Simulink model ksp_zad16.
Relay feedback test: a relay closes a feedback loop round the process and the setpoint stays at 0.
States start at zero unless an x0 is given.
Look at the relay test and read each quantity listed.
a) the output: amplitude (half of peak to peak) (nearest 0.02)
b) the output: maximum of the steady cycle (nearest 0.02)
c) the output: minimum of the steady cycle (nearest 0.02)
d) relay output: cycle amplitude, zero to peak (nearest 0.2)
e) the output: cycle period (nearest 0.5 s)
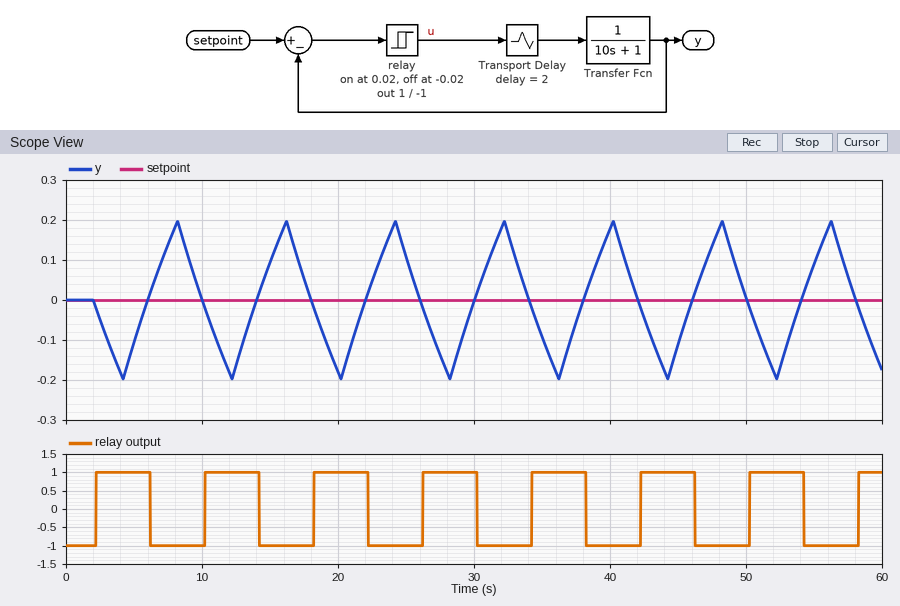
0.20
0.20
-0.20
1.0
8.0 s
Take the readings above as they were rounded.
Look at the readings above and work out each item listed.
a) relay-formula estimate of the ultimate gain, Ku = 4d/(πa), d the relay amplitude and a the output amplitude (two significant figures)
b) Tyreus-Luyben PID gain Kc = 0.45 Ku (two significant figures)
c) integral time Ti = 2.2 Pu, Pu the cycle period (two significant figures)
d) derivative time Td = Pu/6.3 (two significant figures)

6.4
2.9
18 s
1.3 s
